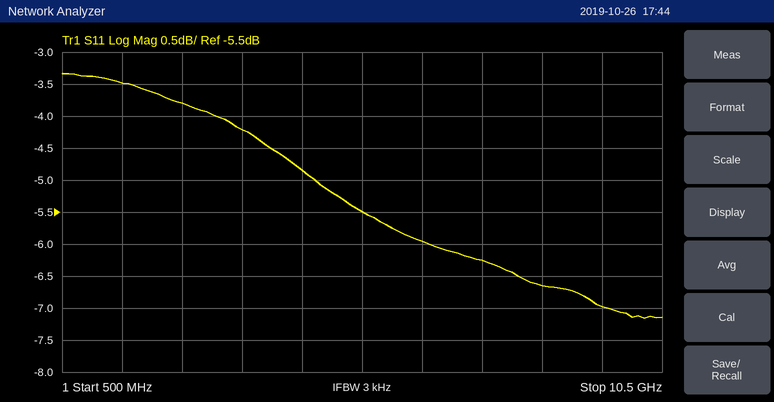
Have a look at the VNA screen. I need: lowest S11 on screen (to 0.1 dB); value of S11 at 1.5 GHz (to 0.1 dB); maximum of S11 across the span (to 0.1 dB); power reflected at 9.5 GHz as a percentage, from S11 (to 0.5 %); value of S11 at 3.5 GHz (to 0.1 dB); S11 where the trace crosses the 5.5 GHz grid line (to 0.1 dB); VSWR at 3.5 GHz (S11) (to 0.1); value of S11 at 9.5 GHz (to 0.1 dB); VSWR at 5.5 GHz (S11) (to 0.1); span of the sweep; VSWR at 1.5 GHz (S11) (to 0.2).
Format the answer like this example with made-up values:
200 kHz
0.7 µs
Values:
-7.2 dB
-3.5 dB
-3.3 dB
20.0 %
-4.2 dB
-5.5 dB
4.2
-7.0 dB
3.3
10 GHz
5.0
